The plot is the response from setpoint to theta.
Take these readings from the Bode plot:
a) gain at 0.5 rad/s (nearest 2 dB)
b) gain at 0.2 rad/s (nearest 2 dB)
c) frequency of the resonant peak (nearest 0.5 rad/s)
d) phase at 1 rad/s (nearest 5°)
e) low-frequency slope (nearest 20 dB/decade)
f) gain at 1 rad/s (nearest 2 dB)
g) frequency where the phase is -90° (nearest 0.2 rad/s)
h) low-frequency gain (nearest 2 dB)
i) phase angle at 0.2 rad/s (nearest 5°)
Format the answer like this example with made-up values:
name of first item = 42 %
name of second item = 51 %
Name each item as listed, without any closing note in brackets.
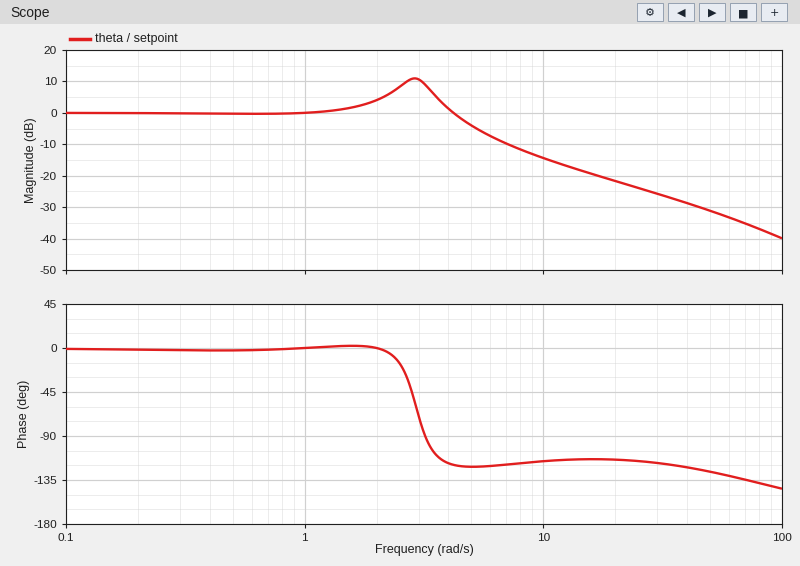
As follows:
gain at 0.5 rad/s = 0 dB
gain at 0.2 rad/s = 0 dB
frequency of the resonant peak = 3.0 rad/s
phase at 1 rad/s = 0°
low-frequency slope = 0 dB/decade
gain at 1 rad/s = 0 dB
frequency where the phase is -90° = 3.2 rad/s
low-frequency gain = 0 dB
phase angle at 0.2 rad/s = 0°
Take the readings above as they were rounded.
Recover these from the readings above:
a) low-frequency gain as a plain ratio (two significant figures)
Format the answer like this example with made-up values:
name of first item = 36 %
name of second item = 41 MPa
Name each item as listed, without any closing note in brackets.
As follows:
low-frequency gain as a plain ratio = 1.0
